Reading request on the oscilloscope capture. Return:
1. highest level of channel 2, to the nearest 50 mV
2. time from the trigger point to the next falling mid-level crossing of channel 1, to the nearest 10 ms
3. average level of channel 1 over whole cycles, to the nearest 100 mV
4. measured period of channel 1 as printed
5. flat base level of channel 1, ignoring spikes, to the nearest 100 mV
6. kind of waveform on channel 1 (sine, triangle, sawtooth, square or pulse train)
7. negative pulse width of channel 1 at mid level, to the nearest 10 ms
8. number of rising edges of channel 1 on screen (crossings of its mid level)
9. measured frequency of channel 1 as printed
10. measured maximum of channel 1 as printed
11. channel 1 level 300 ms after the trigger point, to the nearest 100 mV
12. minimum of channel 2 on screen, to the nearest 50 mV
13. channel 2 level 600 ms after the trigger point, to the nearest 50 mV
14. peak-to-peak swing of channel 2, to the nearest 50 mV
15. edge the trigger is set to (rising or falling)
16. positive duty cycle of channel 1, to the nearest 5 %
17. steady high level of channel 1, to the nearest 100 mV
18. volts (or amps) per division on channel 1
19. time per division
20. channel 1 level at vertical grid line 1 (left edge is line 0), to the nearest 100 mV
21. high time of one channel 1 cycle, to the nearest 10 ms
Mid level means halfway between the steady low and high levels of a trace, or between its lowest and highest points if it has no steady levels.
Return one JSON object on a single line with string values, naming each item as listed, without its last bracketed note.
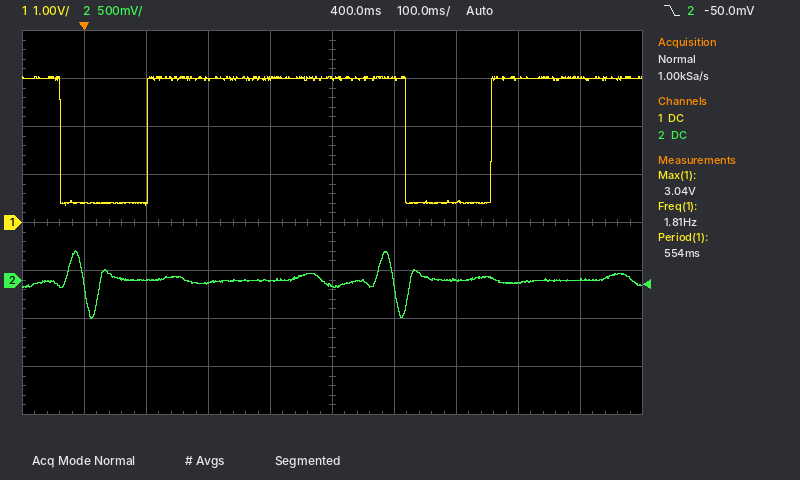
{"highest level of channel 2, to the nearest 50 mV": "300 mV", "time from the trigger point to the next falling mid-level crossing of channel 1, to the nearest 10 ms": "520 ms", "average level of channel 1 over whole cycles, to the nearest 100 mV": "2.4 V", "measured period of channel 1 as printed": "554 ms", "flat base level of channel 1, ignoring spikes, to the nearest 100 mV": "400 mV", "kind of waveform on channel 1": "pulse train", "negative pulse width of channel 1 at mid level, to the nearest 10 ms": "140 ms", "number of rising edges of channel 1 on screen": "2", "measured frequency of channel 1 as printed": "1.81 Hz", "measured maximum of channel 1 as printed": "3.04 V", "channel 1 level 300 ms after the trigger point, to the nearest 100 mV": "3.0 V", "minimum of channel 2 on screen, to the nearest 50 mV": "-400 mV", "channel 2 level 600 ms after the trigger point, to the nearest 50 mV": "0 mV", "peak-to-peak swing of channel 2, to the nearest 50 mV": "700 mV", "edge the trigger is set to": "falling", "positive duty cycle of channel 1, to the nearest 5 %": "75 %", "steady high level of channel 1, to the nearest 100 mV": "3.0 V", "volts (or amps) per division on channel 1": "1 V", "time per division": "100 ms", "channel 1 level at vertical grid line 1 (left edge is line 0), to the nearest 100 mV": "400 mV", "high time of one channel 1 cycle, to the nearest 10 ms": "420 ms"}
